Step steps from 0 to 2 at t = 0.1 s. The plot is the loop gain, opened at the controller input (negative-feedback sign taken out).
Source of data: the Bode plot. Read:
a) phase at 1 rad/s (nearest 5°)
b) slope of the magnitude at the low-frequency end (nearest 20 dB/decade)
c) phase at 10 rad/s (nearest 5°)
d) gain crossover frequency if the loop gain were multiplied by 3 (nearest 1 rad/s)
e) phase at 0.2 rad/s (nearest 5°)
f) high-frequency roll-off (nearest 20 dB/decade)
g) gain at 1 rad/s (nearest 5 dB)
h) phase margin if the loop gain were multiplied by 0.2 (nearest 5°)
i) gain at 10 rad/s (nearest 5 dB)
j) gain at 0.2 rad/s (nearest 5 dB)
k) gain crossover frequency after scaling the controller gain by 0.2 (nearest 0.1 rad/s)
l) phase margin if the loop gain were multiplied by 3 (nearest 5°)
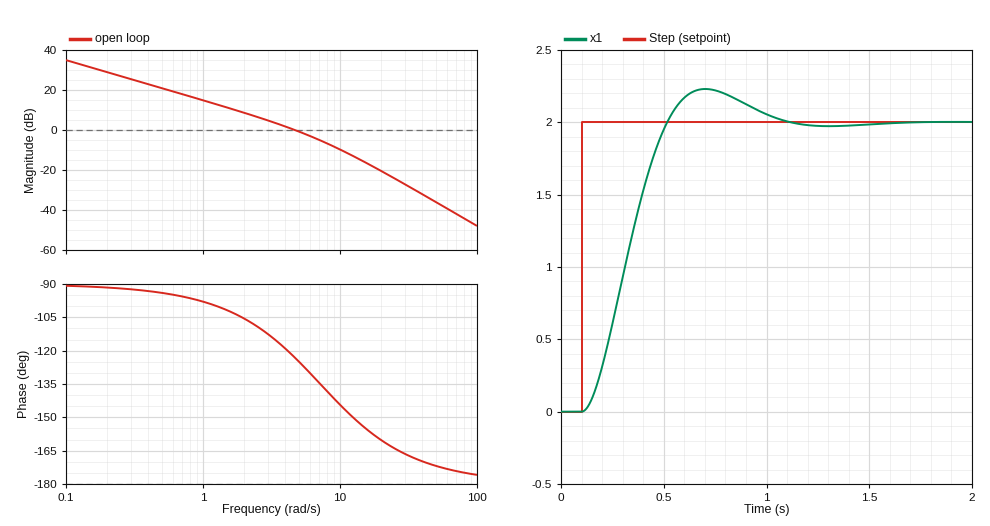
-100°
-20 dB/decade
-145°
10 rad/s
-90°
-40 dB/decade
15 dB
80°
-10 dB
30 dB
1.1 rad/s
35°
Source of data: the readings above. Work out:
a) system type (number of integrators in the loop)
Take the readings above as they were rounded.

1
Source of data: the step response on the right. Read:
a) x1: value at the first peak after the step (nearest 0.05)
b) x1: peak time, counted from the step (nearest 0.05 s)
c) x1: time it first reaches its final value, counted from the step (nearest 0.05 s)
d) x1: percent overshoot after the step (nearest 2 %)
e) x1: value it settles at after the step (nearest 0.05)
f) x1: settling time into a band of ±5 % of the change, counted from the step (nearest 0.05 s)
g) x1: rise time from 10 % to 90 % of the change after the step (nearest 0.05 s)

2.25
0.60 s
0.40 s
12 %
2.00
0.85 s
0.30 s
